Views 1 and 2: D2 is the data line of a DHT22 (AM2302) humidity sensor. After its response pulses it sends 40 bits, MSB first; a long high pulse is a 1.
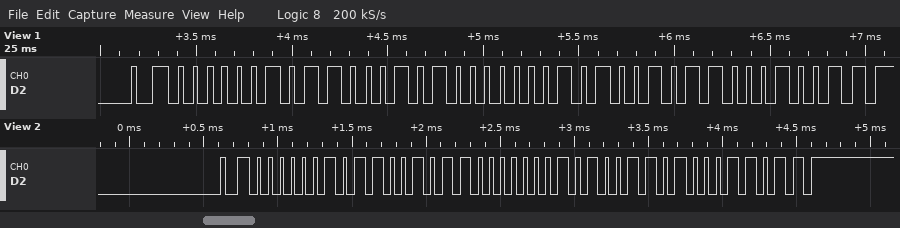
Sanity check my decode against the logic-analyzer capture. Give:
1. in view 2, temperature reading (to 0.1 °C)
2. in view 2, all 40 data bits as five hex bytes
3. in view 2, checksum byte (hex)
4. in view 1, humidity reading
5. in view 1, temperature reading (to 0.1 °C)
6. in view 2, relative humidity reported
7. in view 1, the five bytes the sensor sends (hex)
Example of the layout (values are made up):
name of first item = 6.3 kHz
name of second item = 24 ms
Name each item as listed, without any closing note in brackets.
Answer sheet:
in view 2, temperature reading = 33.3 °C
in view 2, all 40 data bits as five hex bytes = 02 CB 01 4D 1B
in view 2, checksum byte = 0x1B
in view 1, humidity reading = 70.9 %
in view 1, temperature reading = 33.1 °C
in view 2, relative humidity reported = 71.5 %
in view 1, the five bytes the sensor sends = 02 C5 01 4B 13
